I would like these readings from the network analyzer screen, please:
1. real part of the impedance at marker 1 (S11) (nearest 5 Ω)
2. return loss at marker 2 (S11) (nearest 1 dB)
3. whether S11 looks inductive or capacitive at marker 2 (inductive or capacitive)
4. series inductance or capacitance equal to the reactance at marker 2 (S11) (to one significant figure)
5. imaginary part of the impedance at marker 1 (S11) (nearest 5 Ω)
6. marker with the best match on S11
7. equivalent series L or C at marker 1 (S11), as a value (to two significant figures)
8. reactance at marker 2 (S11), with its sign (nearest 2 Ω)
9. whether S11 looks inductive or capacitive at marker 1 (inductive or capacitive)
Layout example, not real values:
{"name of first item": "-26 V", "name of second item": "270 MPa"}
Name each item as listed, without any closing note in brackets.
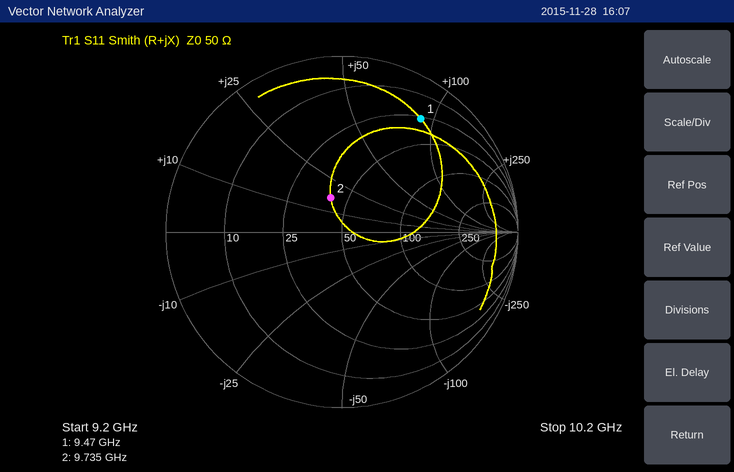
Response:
{"real part of the impedance at marker 1 (S11)": "25 Ω", "return loss at marker 2 (S11)": "14 dB", "whether S11 looks inductive or capacitive at marker 2": "inductive", "series inductance or capacitance equal to the reactance at marker 2 (S11)": "300 pH", "imaginary part of the impedance at marker 1 (S11)": "+90 Ω", "marker with the best match on S11": "marker 2", "equivalent series L or C at marker 1 (S11), as a value": "1.5 nH", "reactance at marker 2 (S11), with its sign": "+16 Ω", "whether S11 looks inductive or capacitive at marker 1": "inductive"}
